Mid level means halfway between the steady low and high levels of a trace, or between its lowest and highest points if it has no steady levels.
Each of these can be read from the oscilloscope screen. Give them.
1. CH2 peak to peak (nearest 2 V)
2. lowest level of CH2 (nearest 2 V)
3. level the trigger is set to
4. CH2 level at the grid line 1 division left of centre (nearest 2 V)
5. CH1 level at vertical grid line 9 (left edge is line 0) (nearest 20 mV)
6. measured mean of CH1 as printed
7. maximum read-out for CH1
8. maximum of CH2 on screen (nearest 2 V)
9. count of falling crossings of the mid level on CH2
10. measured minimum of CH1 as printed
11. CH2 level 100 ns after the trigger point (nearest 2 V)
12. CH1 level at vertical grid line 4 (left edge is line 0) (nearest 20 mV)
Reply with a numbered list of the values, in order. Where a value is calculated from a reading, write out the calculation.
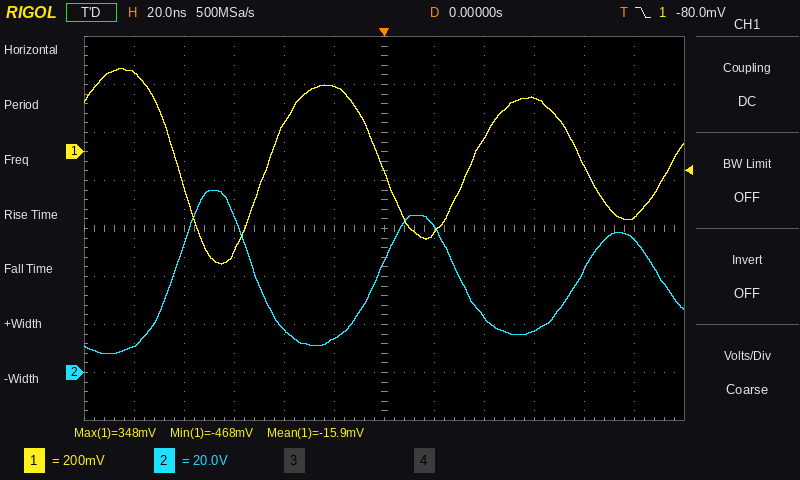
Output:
1. 76 V − (8 V) = 68 V
2. 8 V
3. -80.0 mV
4. 14 V
5. 220 mV
6. -15.9 mV
7. 348 mV
8. 76 V
9. 3
10. -468 mV
11. 56 V
12. 120 mV
